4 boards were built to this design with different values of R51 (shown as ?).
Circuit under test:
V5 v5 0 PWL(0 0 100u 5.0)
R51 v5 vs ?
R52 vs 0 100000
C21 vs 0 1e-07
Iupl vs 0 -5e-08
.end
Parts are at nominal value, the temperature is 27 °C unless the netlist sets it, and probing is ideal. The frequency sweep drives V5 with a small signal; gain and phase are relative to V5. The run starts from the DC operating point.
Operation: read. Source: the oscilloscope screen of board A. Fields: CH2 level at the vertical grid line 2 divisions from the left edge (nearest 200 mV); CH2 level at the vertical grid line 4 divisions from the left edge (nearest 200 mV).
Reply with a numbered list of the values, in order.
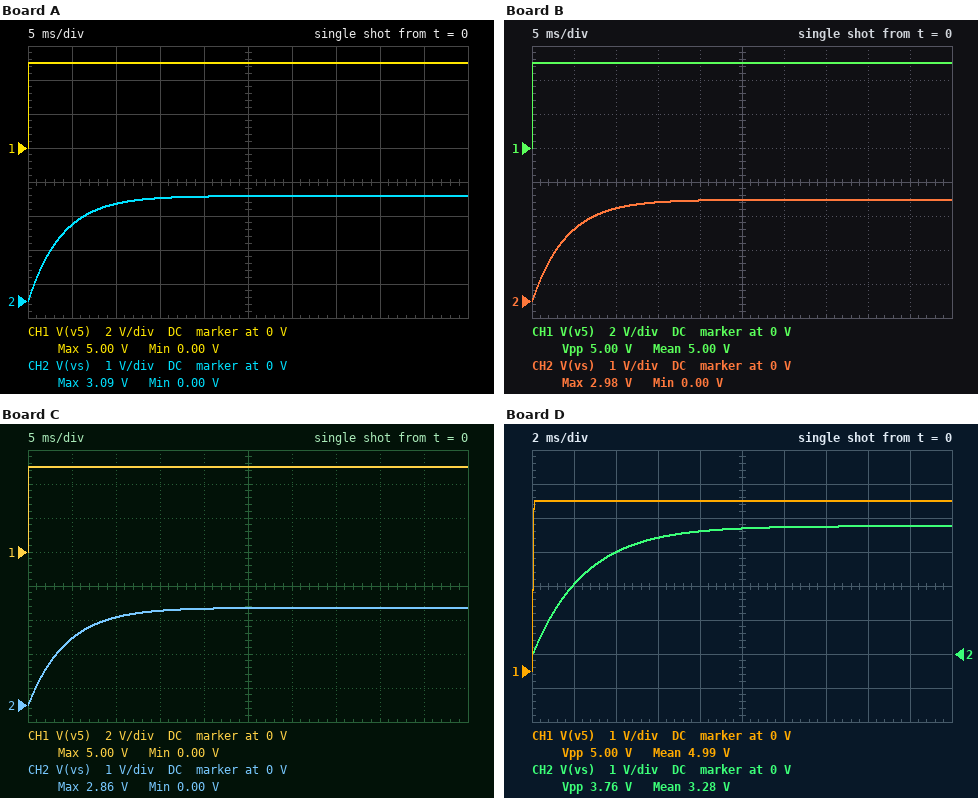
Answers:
1. 2.8 V
2. 3.0 V
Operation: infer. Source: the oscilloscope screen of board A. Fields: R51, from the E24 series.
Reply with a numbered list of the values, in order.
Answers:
1. 62 kΩ
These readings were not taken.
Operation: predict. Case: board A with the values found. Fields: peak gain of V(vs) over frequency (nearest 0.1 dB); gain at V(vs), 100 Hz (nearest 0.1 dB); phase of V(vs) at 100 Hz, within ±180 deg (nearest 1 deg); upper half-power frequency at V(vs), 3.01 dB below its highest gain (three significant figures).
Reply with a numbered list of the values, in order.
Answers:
1. -4.2 dB
2. -12.5 dB
3. -67 deg
4. 41.6 Hz
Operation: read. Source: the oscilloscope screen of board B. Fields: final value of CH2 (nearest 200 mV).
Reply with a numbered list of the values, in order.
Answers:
1. 3.0 V
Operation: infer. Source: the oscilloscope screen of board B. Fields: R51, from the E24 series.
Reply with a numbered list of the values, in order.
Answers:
1. 68 kΩ
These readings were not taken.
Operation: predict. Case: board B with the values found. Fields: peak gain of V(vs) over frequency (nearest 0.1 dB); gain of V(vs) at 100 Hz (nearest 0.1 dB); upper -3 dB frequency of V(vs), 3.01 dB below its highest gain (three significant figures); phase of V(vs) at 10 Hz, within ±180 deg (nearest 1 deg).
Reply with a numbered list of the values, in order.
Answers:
1. -4.5 dB
2. -13.2 dB
3. 39.3 Hz
4. -14 deg
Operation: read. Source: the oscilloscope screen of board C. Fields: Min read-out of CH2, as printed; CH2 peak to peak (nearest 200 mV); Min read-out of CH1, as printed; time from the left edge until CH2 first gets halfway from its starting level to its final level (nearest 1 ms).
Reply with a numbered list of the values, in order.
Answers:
1. 0.00 V
2. 2.8 V
3. 0.00 V
4. 3 ms
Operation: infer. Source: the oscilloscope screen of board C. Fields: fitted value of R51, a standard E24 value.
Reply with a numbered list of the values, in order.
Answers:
1. 75 kΩ
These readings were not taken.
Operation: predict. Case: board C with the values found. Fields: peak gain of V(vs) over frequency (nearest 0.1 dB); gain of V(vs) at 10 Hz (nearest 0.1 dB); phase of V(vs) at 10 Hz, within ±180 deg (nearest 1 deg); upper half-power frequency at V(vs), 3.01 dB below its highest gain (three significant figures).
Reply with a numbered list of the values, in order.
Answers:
1. -4.9 dB
2. -5.2 dB
3. -15 deg
4. 37.1 Hz
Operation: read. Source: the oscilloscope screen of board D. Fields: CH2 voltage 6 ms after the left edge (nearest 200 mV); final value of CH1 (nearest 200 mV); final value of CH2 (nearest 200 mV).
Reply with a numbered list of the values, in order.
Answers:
1. 3.4 V
2. 5.0 V
3. 3.8 V
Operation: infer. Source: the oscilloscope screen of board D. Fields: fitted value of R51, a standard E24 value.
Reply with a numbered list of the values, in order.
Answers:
1. 33 kΩ
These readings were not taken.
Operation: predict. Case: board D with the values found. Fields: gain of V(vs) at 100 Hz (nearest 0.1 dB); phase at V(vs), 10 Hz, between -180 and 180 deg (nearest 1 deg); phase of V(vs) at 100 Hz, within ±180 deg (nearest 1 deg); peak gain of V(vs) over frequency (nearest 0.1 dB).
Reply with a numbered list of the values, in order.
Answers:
1. -7.8 dB
2. -9 deg
3. -57 deg
4. -2.5 dB
